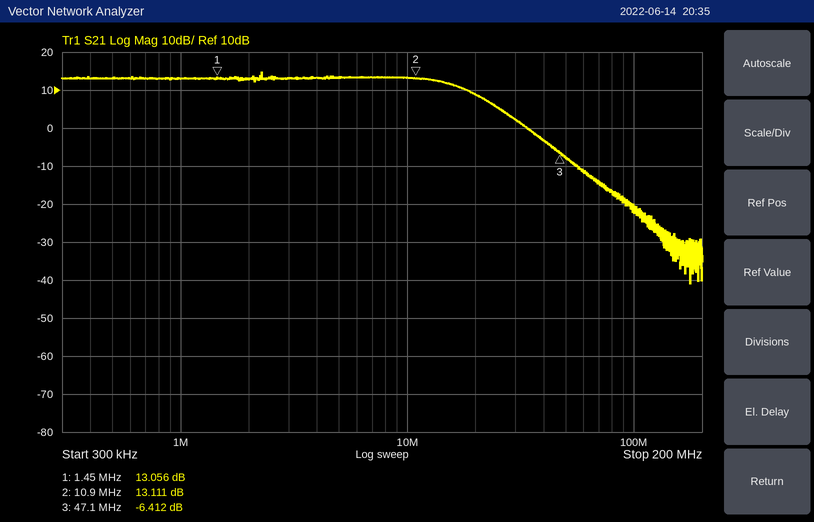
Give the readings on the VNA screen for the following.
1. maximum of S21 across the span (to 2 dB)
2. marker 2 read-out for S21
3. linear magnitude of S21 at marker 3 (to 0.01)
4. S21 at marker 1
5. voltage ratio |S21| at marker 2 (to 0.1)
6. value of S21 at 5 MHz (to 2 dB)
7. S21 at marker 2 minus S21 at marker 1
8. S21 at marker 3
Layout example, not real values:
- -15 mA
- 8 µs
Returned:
- 14 dB
- 13.111 dB
- 0.48
- 13.056 dB
- 4.5
- 14 dB
- 0.055 dB
- -6.412 dB
